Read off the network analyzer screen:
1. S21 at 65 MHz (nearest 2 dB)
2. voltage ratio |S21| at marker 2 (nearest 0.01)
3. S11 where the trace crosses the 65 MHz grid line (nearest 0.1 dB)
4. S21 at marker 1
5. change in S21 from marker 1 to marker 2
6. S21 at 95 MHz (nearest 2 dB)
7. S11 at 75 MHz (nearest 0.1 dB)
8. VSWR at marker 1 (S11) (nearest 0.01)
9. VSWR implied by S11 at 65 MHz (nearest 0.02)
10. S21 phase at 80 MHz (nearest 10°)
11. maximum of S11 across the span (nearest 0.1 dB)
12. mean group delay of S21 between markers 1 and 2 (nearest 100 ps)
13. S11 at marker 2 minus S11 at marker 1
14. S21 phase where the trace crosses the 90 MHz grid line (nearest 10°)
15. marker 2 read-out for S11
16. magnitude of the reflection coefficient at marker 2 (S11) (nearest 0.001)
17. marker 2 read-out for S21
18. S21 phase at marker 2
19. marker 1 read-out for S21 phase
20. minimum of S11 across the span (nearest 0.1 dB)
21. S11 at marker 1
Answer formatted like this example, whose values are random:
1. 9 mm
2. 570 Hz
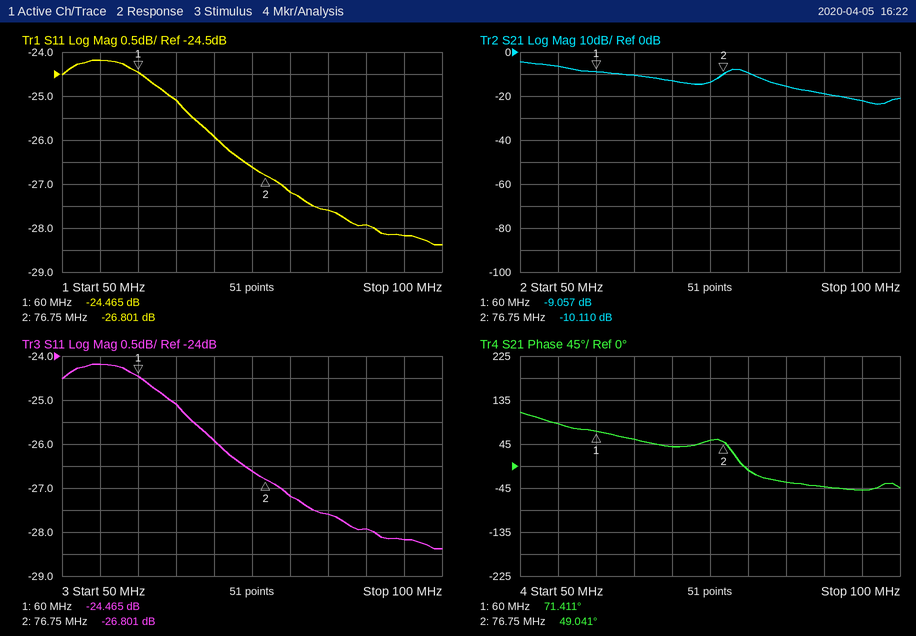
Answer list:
1. -10 dB
2. 0.31
3. -25.1 dB
4. -9.057 dB
5. -1.053 dB
6. -22 dB
7. -26.6 dB
8. 1.13
9. 1.12
10. -10°
11. -24.2 dB
12. 3.7 ns
13. -2.336 dB
14. -40°
15. -26.801 dB
16. 0.046
17. -10.110 dB
18. 49.041°
19. 71.411°
20. -28.4 dB
21. -24.465 dB
